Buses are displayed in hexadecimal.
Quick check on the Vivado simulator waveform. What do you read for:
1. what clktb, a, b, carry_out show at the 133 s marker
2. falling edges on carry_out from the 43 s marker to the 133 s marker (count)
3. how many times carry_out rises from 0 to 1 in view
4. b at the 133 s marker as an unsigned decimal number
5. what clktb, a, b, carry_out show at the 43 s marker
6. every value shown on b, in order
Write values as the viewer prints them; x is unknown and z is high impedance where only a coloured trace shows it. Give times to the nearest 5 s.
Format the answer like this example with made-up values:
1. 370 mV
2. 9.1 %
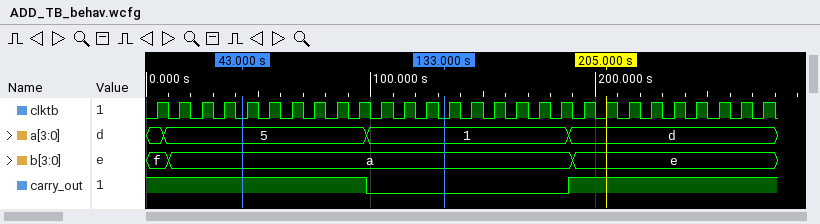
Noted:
1. clktb=0, a=1, b=a, carry_out=0
2. 1
3. 1
4. 10
5. clktb=0, a=5, b=a, carry_out=1
6. f, a, e
